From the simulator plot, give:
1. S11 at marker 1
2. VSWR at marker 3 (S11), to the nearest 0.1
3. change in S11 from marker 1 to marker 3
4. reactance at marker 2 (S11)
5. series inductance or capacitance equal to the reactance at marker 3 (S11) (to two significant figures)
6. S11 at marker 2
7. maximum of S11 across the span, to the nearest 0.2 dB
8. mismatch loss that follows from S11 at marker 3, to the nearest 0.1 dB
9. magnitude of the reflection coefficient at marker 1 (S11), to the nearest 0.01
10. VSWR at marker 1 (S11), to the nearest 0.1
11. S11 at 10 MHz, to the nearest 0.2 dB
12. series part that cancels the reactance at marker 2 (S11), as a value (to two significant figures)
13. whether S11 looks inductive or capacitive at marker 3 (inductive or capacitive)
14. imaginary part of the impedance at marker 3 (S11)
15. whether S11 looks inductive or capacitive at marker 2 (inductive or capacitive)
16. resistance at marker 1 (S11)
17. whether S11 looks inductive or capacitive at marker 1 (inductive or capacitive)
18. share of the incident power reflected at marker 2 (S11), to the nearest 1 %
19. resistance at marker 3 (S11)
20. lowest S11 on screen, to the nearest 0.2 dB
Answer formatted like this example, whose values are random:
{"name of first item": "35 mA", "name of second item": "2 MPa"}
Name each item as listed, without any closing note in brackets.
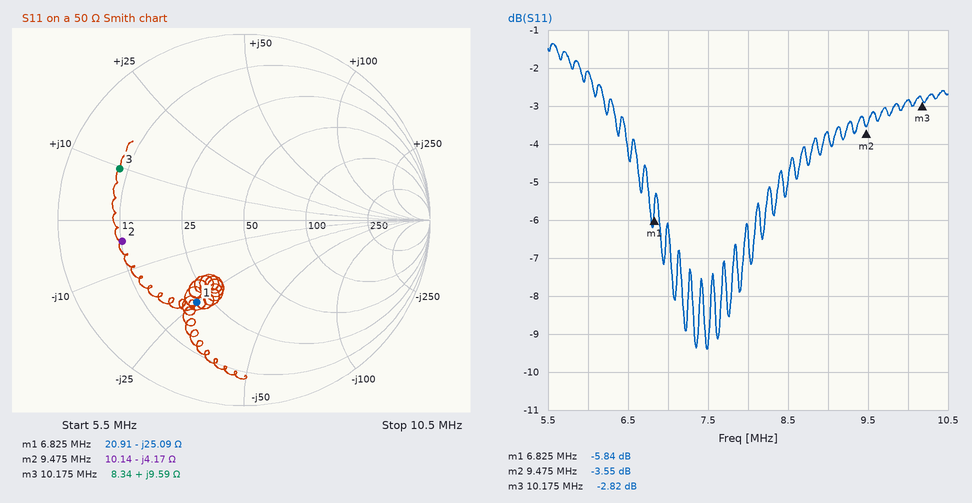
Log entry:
{"S11 at marker 1": "-5.84 dB", "VSWR at marker 3 (S11), to the nearest 0.1": "6.2", "change in S11 from marker 1 to marker 3": "3.02 dB", "reactance at marker 2": "-4.17 Ω", "series inductance or capacitance equal to the reactance at marker 3 (S11)": "150 nH", "S11 at marker 2": "-3.55 dB", "maximum of S11 across the span, to the nearest 0.2 dB": "-1.4 dB", "mismatch loss that follows from S11 at marker 3, to the nearest 0.1 dB": "3.2 dB", "magnitude of the reflection coefficient at marker 1 (S11), to the nearest 0.01": "0.51", "VSWR at marker 1 (S11), to the nearest 0.1": "3.1", "S11 at 10 MHz, to the nearest 0.2 dB": "-2.8 dB", "series part that cancels the reactance at marker 2 (S11), as a value": "70 nH", "whether S11 looks inductive or capacitive at marker 3": "inductive", "imaginary part of the impedance at marker 3": "+9.59 Ω", "whether S11 looks inductive or capacitive at marker 2": "capacitive", "resistance at marker 1": "20.91 Ω", "whether S11 looks inductive or capacitive at marker 1": "capacitive", "share of the incident power reflected at marker 2 (S11), to the nearest 1 %": "44 %", "resistance at marker 3": "8.34 Ω", "lowest S11 on screen, to the nearest 0.2 dB": "-9.4 dB"}
